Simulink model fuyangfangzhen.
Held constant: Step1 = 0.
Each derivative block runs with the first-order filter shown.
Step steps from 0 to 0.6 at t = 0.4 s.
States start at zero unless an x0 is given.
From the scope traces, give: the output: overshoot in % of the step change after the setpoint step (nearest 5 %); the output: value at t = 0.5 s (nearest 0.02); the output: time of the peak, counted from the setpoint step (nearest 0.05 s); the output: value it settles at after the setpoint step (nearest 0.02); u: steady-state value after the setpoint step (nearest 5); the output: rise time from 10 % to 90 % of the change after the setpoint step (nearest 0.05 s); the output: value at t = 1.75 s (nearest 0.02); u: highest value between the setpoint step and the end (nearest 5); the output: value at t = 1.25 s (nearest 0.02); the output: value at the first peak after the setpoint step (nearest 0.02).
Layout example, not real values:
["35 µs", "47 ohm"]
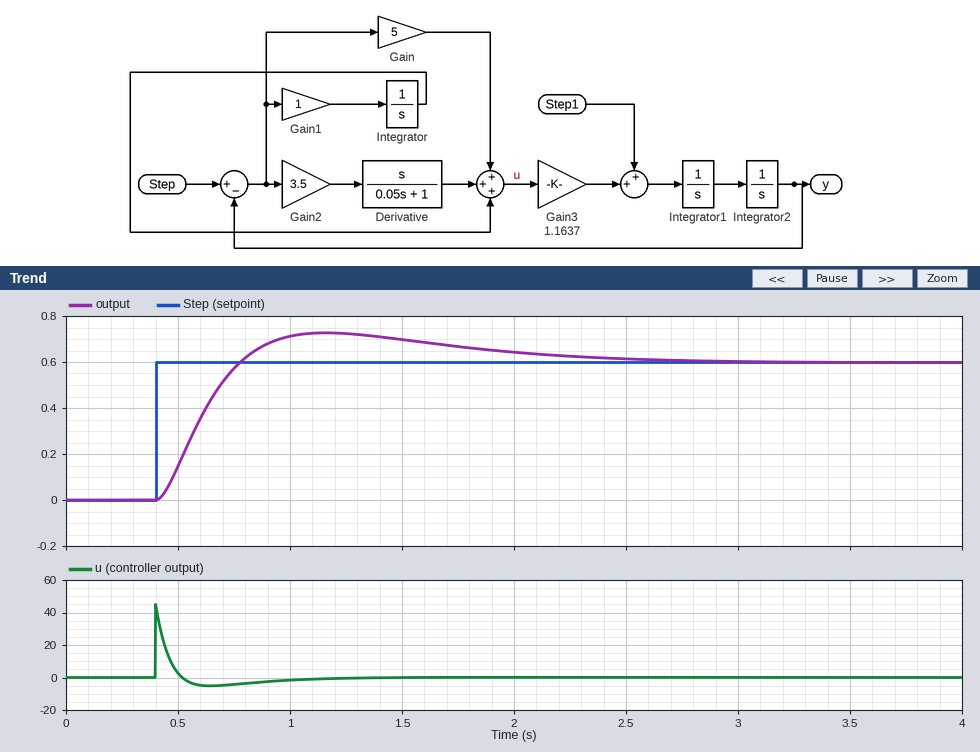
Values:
["20 %", "0.14", "0.75 s", "0.60", "0", "0.25 s", "0.66", "45", "0.72", "0.72"]
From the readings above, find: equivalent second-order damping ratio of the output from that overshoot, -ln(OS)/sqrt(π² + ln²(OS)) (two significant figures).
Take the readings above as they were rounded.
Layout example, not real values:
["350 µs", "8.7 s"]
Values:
["0.46"]
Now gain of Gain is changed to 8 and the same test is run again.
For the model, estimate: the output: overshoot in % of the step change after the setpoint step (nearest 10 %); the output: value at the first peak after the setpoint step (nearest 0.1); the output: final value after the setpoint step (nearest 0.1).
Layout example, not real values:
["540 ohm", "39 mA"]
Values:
["30 %", "0.8", "0.6"]
